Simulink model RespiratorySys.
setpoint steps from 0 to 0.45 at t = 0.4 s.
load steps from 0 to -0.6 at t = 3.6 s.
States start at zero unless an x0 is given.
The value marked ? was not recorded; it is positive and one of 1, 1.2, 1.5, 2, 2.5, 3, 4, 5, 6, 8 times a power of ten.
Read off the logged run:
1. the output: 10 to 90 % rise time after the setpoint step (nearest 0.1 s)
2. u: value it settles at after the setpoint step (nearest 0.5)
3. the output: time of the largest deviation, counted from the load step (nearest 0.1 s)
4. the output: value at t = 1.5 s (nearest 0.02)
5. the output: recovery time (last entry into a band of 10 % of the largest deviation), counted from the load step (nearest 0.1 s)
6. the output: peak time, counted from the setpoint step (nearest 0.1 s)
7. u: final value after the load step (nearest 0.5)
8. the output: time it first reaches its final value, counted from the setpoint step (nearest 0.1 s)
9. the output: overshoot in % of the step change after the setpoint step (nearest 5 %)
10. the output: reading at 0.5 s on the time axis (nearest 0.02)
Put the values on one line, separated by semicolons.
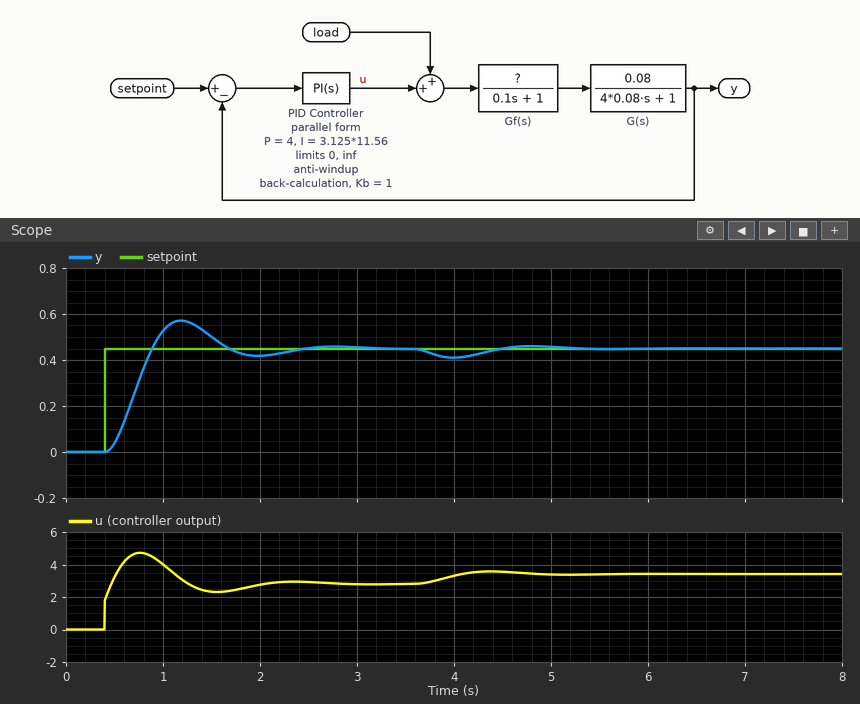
0.3 s; 3.0; 0.4 s; 0.50; 1.5 s; 0.8 s; 3.5; 0.5 s; 25 %; 0.04
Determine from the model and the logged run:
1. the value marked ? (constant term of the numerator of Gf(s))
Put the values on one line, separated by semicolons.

2
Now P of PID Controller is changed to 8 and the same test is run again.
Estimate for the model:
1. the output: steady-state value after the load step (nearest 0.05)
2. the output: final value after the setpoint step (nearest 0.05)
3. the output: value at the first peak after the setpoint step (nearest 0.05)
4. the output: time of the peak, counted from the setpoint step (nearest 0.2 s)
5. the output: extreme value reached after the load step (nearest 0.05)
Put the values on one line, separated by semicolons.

0.45; 0.45; 0.50; 0.6 s; 0.40
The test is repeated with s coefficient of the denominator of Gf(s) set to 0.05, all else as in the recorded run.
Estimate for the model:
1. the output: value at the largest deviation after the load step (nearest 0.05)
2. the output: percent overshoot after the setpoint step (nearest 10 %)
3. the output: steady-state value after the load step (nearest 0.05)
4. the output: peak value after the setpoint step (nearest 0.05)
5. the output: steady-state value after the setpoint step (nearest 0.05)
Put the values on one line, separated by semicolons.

0.40; 20 %; 0.45; 0.55; 0.45
